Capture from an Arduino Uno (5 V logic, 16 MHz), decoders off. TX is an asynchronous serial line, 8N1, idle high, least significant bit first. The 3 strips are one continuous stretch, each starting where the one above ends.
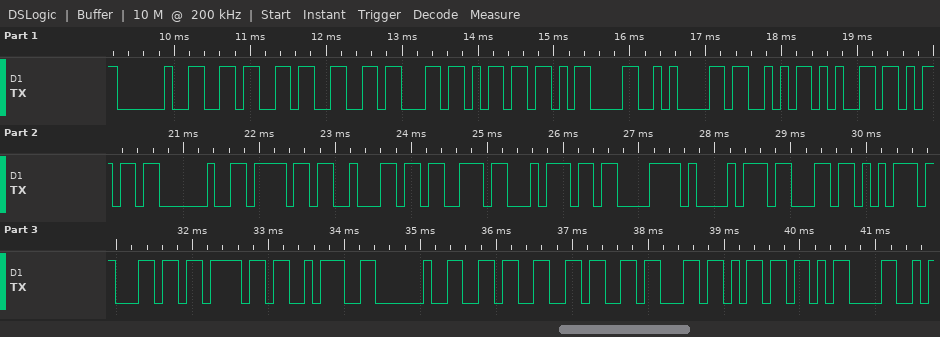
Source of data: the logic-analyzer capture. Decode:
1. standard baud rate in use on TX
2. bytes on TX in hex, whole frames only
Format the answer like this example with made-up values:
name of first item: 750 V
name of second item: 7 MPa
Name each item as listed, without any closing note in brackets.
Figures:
standard baud rate in use on TX: 9600 baud
bytes on TX in hex, whole frames only: 0x20 0x36 0x33 0x63 0x6D 0x0D 0x0A 0x53 0x65 0x6D 0x20 0x6F 0x62 0x73 0x74 0xC3 0xA1 0x63 0x75 0x6C 0x6F 0x3A 0x20 0x36 0x36 0x63 0x6D 0x0D
